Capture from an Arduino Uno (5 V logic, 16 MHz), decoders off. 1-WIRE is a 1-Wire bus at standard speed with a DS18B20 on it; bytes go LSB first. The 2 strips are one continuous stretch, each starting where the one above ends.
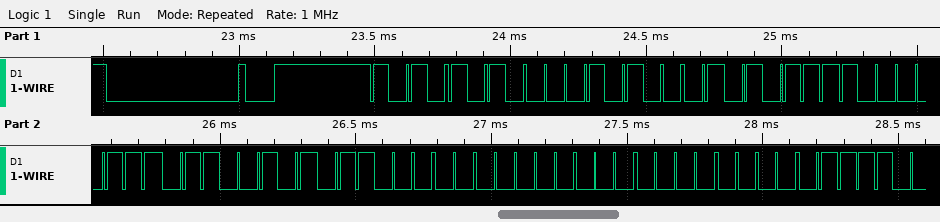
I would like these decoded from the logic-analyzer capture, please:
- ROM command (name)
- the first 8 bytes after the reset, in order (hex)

Match ROM
55 28 EA E1 A6 06 00 00
